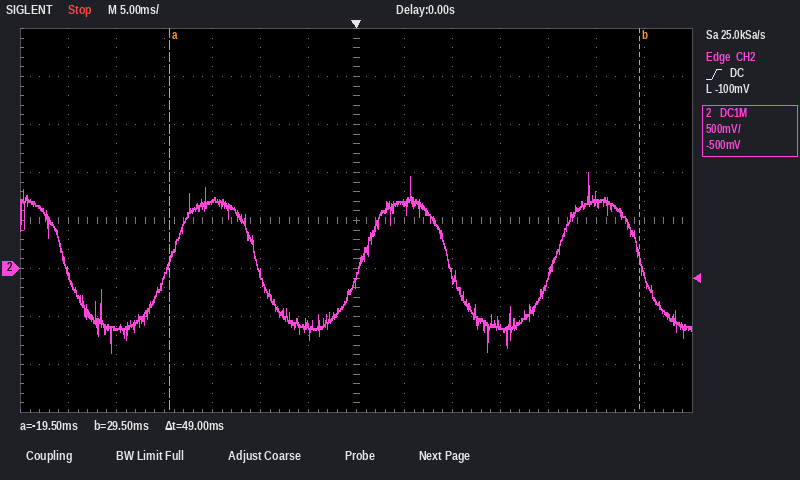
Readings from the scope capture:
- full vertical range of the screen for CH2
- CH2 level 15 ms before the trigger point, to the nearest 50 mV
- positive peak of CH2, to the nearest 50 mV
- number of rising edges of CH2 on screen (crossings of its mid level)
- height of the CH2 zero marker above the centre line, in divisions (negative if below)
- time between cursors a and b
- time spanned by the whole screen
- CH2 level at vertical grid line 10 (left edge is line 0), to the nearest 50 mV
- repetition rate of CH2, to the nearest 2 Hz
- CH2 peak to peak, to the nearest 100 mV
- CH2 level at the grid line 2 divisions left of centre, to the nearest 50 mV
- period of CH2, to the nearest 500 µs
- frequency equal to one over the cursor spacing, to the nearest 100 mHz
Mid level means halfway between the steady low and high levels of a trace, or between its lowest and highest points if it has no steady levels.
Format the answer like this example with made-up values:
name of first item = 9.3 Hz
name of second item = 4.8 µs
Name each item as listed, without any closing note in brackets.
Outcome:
full vertical range of the screen for CH2 = 4 V
CH2 level 15 ms before the trigger point, to the nearest 50 mV = 700 mV
positive peak of CH2, to the nearest 50 mV = 1.00 V
number of rising edges of CH2 on screen = 3
height of the CH2 zero marker above the centre line, in divisions = -1.0 div
time between cursors a and b = 49 ms
time spanned by the whole screen = 70 ms
CH2 level at vertical grid line 10 (left edge is line 0), to the nearest 50 mV = -600 mV
repetition rate of CH2, to the nearest 2 Hz = 50 Hz
CH2 peak to peak, to the nearest 100 mV = 1.90 V
CH2 level at the grid line 2 divisions left of centre, to the nearest 50 mV = -50 mV
period of CH2, to the nearest 500 µs = 20.0 ms
frequency equal to one over the cursor spacing, to the nearest 100 mHz = 20.4 Hz
